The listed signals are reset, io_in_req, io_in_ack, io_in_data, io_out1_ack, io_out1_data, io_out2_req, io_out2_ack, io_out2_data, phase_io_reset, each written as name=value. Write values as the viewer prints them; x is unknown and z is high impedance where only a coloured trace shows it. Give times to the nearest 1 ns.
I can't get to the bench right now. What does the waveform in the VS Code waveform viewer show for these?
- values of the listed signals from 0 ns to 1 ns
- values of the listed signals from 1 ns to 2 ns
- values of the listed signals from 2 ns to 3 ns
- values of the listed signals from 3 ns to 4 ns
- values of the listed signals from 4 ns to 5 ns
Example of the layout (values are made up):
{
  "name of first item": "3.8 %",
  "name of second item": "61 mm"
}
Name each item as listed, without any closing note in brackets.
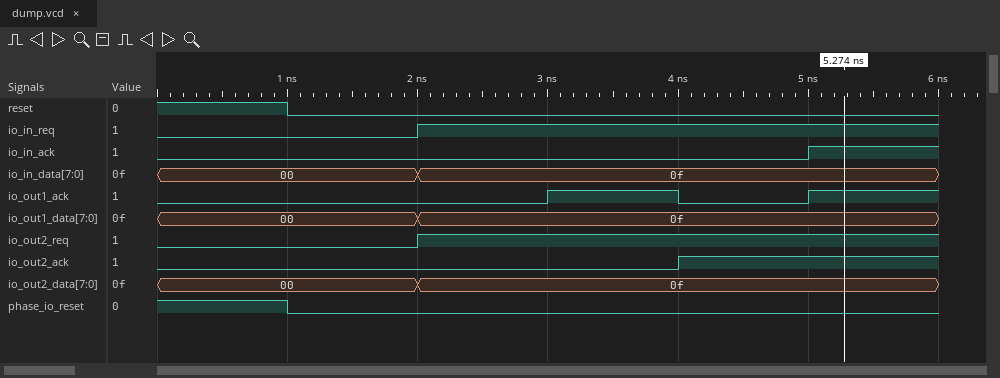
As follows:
{
  "values of the listed signals from 0 ns to 1 ns": "reset=1, io_in_req=0, io_in_ack=0, io_in_data=00, io_out1_ack=0, io_out1_data=00, io_out2_req=0, io_out2_ack=0, io_out2_data=00, phase_io_reset=1",
  "values of the listed signals from 1 ns to 2 ns": "reset=0, io_in_req=0, io_in_ack=0, io_in_data=00, io_out1_ack=0, io_out1_data=00, io_out2_req=0, io_out2_ack=0, io_out2_data=00, phase_io_reset=0",
  "values of the listed signals from 2 ns to 3 ns": "reset=0, io_in_req=1, io_in_ack=0, io_in_data=0f, io_out1_ack=0, io_out1_data=0f, io_out2_req=1, io_out2_ack=0, io_out2_data=0f, phase_io_reset=0",
  "values of the listed signals from 3 ns to 4 ns": "reset=0, io_in_req=1, io_in_ack=0, io_in_data=0f, io_out1_ack=1, io_out1_data=0f, io_out2_req=1, io_out2_ack=0, io_out2_data=0f, phase_io_reset=0",
  "values of the listed signals from 4 ns to 5 ns": "reset=0, io_in_req=1, io_in_ack=0, io_in_data=0f, io_out1_ack=0, io_out1_data=0f, io_out2_req=1, io_out2_ack=1, io_out2_data=0f, phase_io_reset=0"
}
